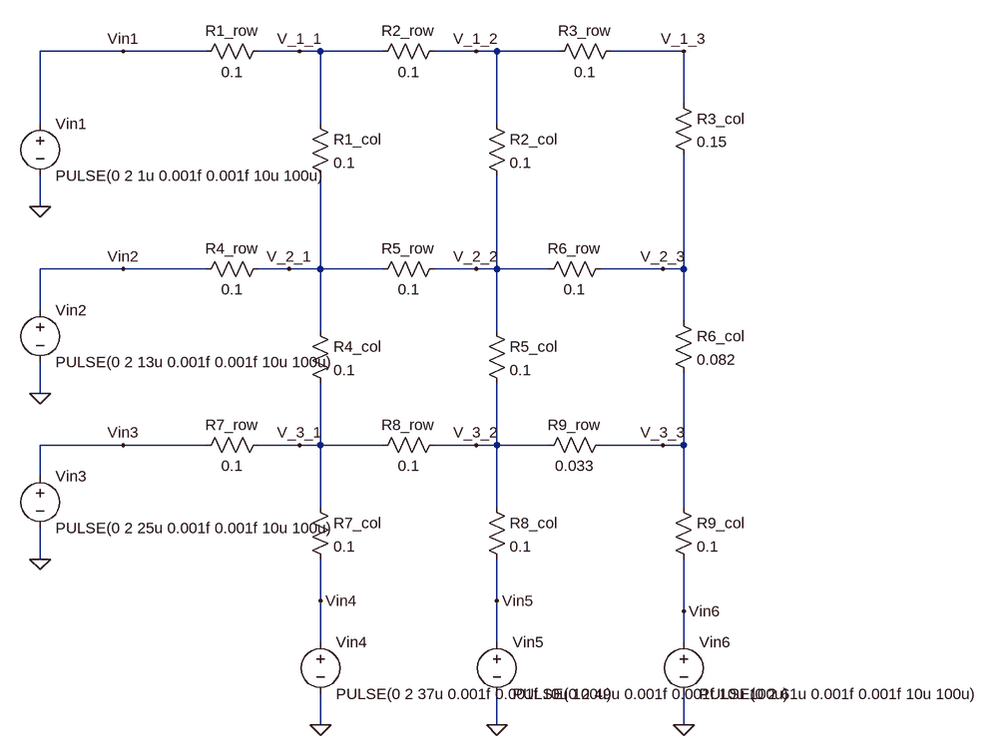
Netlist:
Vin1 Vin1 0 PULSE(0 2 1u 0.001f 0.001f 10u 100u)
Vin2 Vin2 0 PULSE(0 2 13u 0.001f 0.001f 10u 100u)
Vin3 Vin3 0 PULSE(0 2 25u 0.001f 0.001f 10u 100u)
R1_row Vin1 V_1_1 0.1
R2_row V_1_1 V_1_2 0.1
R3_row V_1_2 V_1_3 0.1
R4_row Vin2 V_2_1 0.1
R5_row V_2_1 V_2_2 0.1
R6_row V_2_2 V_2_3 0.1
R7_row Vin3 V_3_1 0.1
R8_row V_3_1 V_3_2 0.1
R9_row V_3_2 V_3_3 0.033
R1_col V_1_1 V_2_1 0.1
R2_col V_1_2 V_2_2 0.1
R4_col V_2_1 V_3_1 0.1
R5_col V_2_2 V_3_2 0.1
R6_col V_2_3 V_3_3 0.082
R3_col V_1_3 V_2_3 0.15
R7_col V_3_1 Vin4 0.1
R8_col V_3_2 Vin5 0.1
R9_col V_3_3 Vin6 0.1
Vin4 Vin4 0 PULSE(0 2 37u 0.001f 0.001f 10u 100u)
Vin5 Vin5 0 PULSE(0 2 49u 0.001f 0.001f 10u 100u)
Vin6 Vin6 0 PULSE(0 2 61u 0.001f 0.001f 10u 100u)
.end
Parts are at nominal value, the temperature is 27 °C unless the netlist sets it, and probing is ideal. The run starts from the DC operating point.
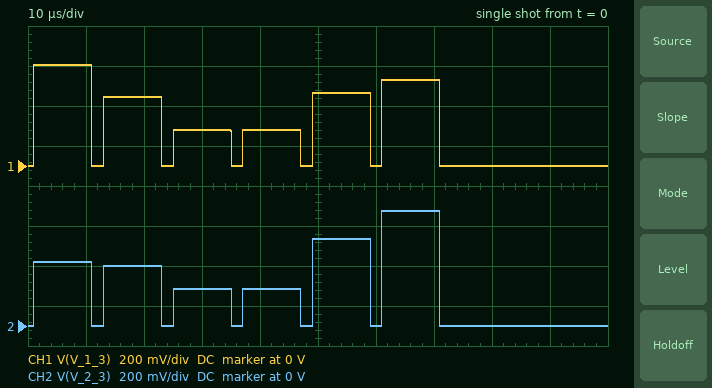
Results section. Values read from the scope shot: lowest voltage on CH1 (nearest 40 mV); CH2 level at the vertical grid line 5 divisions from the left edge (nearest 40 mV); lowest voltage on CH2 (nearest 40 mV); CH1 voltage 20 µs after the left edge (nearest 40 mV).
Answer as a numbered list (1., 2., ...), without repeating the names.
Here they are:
1. 0 V
2. 440 mV
3. 0 V
4. 360 mV
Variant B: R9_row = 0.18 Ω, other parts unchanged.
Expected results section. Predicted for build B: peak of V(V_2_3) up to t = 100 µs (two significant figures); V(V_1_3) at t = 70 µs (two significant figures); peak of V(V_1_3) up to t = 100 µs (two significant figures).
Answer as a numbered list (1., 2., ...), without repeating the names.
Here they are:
1. 710 mV
2. 500 mV
3. 500 mV
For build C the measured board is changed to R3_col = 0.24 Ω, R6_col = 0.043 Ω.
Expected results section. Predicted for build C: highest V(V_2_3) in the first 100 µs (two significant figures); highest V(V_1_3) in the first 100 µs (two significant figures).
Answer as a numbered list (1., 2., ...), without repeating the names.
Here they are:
1. 650 mV
2. 520 mV
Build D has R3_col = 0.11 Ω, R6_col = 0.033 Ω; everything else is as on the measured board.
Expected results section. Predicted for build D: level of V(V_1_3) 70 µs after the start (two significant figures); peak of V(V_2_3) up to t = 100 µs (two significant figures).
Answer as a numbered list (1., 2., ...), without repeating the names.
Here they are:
1. 510 mV
2. 660 mV
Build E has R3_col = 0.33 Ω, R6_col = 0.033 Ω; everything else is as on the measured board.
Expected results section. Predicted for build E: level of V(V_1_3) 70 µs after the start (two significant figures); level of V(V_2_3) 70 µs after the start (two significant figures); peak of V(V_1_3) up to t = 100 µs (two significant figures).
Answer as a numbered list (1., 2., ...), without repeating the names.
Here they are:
1. 420 mV
2. 680 mV
3. 540 mV
